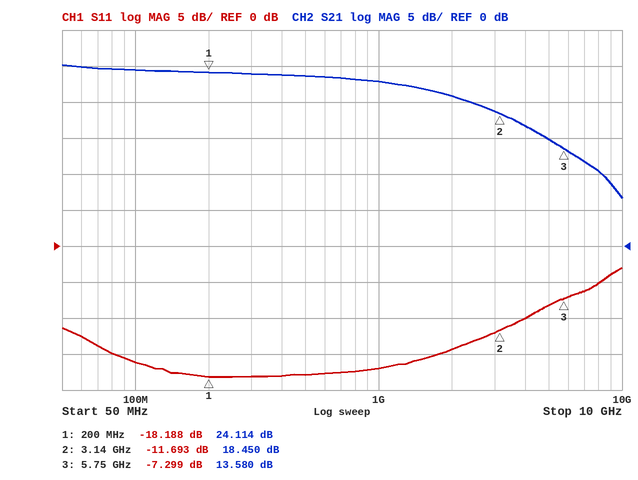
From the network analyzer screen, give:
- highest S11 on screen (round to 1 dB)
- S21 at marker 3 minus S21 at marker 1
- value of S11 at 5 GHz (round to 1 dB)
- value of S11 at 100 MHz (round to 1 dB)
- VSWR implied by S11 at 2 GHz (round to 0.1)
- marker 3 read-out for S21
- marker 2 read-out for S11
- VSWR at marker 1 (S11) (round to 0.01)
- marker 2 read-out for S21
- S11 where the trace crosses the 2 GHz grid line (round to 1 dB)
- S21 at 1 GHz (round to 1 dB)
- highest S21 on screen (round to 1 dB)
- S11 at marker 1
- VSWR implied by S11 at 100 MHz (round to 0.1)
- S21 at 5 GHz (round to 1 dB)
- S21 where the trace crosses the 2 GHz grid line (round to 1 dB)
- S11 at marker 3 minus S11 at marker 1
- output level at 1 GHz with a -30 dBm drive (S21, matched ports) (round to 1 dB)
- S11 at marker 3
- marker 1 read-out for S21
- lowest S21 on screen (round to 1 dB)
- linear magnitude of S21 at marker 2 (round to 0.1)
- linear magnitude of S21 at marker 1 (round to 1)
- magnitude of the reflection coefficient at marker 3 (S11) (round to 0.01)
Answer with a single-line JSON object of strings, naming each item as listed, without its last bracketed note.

{"highest S11 on screen": "-3 dB", "S21 at marker 3 minus S21 at marker 1": "-10.534 dB", "value of S11 at 5 GHz": "-8 dB", "value of S11 at 100 MHz": "-16 dB", "VSWR implied by S11 at 2 GHz": "1.5", "marker 3 read-out for S21": "13.580 dB", "marker 2 read-out for S11": "-11.693 dB", "VSWR at marker 1 (S11)": "1.28", "marker 2 read-out for S21": "18.450 dB", "S11 where the trace crosses the 2 GHz grid line": "-14 dB", "S21 at 1 GHz": "23 dB", "highest S21 on screen": "25 dB", "S11 at marker 1": "-18.188 dB", "VSWR implied by S11 at 100 MHz": "1.4", "S21 at 5 GHz": "15 dB", "S21 where the trace crosses the 2 GHz grid line": "21 dB", "S11 at marker 3 minus S11 at marker 1": "10.889 dB", "output level at 1 GHz with a -30 dBm drive (S21, matched ports)": "-7 dBm", "S11 at marker 3": "-7.299 dB", "marker 1 read-out for S21": "24.114 dB", "lowest S21 on screen": "7 dB", "linear magnitude of S21 at marker 2": "8.4", "linear magnitude of S21 at marker 1": "16", "magnitude of the reflection coefficient at marker 3 (S11)": "0.43"}
